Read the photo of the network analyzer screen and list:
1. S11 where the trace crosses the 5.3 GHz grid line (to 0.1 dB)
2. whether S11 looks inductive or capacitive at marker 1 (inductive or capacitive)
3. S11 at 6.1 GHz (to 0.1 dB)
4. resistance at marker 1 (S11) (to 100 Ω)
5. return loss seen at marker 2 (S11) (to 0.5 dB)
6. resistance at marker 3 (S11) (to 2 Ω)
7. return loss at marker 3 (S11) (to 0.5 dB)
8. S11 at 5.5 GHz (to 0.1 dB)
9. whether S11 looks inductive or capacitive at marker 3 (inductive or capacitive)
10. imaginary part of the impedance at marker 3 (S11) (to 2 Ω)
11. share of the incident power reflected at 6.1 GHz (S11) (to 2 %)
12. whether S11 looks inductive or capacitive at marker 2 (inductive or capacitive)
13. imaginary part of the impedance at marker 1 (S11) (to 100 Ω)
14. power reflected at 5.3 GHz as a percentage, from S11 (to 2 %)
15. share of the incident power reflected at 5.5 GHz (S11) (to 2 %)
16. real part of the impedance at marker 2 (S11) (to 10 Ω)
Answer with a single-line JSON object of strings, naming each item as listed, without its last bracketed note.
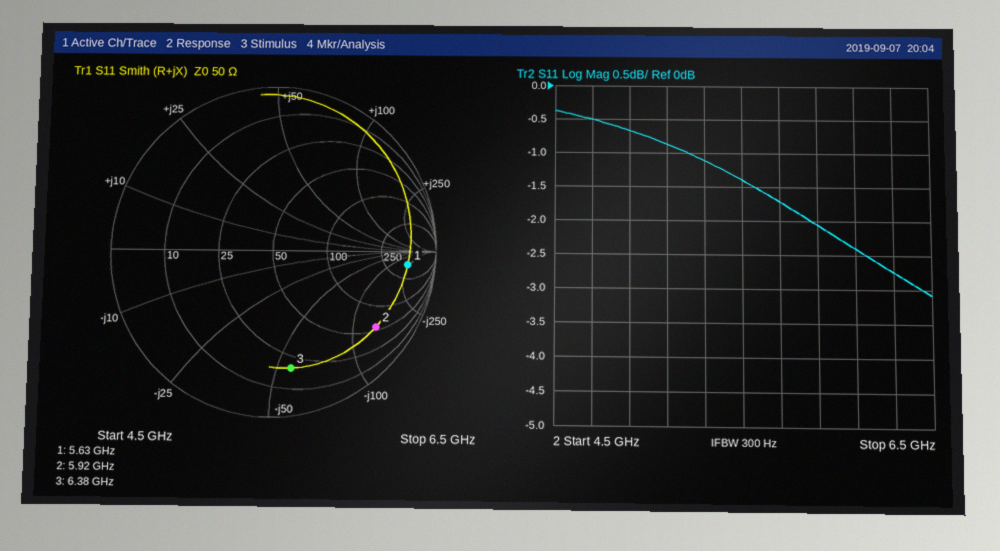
{"S11 where the trace crosses the 5.3 GHz grid line": "-1.1 dB", "whether S11 looks inductive or capacitive at marker 1": "capacitive", "S11 at 6.1 GHz": "-2.4 dB", "resistance at marker 1 (S11)": "400 Ω", "return loss seen at marker 2 (S11)": "2.0 dB", "resistance at marker 3 (S11)": "20 Ω", "return loss at marker 3 (S11)": "3.0 dB", "S11 at 5.5 GHz": "-1.4 dB", "whether S11 looks inductive or capacitive at marker 3": "capacitive", "imaginary part of the impedance at marker 3 (S11)": "-56 Ω", "share of the incident power reflected at 6.1 GHz (S11)": "58 %", "whether S11 looks inductive or capacitive at marker 2": "capacitive", "imaginary part of the impedance at marker 1 (S11)": "-200 Ω", "power reflected at 5.3 GHz as a percentage, from S11": "78 %", "share of the incident power reflected at 5.5 GHz (S11)": "72 %", "real part of the impedance at marker 2 (S11)": "60 Ω"}
